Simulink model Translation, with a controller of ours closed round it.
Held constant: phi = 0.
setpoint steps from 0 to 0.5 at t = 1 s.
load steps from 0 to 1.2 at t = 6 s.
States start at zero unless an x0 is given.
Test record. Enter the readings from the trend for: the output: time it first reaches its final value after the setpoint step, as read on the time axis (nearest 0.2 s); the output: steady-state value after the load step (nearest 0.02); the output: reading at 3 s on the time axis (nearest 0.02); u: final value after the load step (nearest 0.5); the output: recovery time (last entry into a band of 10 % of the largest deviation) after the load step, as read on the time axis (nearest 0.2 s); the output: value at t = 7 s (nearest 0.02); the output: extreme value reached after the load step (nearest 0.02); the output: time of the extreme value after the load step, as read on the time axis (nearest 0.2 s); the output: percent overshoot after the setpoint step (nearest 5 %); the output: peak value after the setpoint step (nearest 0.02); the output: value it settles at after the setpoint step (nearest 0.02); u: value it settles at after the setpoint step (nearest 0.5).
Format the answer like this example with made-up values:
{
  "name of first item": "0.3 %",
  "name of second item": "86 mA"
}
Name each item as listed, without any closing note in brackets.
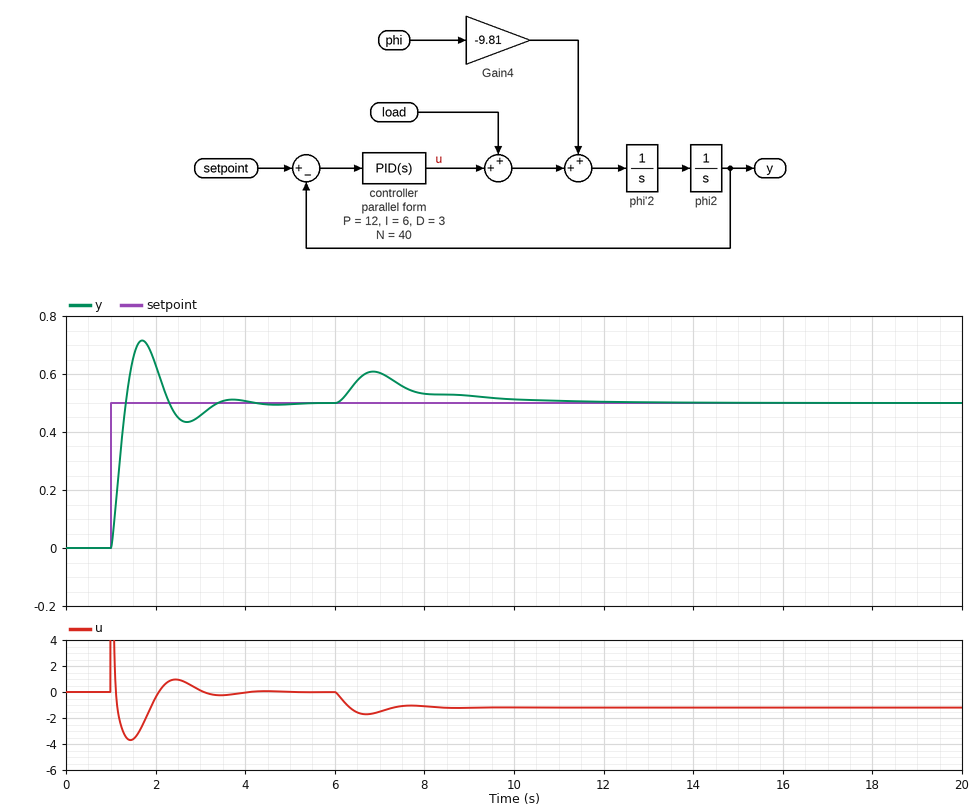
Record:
{
  "the output: time it first reaches its final value after the setpoint step, as read on the time axis": "1.4 s",
  "the output: steady-state value after the load step": "0.50",
  "the output: reading at 3 s on the time axis": "0.46",
  "u: final value after the load step": "-1.0",
  "the output: recovery time (last entry into a band of 10 % of the largest deviation) after the load step, as read on the time axis": "10.2 s",
  "the output: value at t = 7 s": "0.60",
  "the output: extreme value reached after the load step": "0.60",
  "the output: time of the extreme value after the load step, as read on the time axis": "6.8 s",
  "the output: percent overshoot after the setpoint step": "45 %",
  "the output: peak value after the setpoint step": "0.72",
  "the output: value it settles at after the setpoint step": "0.50",
  "u: value it settles at after the setpoint step": "0.0"
}
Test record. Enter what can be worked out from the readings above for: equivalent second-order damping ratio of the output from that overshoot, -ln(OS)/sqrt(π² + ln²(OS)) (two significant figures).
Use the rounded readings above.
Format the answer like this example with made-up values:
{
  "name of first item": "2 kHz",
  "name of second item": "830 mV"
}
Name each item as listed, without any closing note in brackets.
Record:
{
  "equivalent second-order damping ratio of the output from that overshoot, -ln(OS)/sqrt(π² + ln²(OS))": "0.25"
}
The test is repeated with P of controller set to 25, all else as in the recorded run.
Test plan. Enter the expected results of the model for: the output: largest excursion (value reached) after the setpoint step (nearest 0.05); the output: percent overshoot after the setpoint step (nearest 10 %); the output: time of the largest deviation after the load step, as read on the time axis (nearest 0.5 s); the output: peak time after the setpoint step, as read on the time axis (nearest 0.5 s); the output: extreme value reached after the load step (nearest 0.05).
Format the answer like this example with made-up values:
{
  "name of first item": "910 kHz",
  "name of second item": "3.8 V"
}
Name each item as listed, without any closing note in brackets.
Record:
{
  "the output: largest excursion (value reached) after the setpoint step": "0.75",
  "the output: percent overshoot after the setpoint step": "50 %",
  "the output: time of the largest deviation after the load step, as read on the time axis": "6.5 s",
  "the output: peak time after the setpoint step, as read on the time axis": "1.5 s",
  "the output: extreme value reached after the load step": "0.55"
}
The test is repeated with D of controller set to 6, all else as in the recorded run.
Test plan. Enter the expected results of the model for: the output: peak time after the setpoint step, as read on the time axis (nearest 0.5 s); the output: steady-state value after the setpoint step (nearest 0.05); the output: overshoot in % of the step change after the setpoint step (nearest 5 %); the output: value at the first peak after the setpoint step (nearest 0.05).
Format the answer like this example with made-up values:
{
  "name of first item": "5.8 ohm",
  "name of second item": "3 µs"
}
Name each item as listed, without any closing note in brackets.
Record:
{
  "the output: peak time after the setpoint step, as read on the time axis": "1.5 s",
  "the output: steady-state value after the setpoint step": "0.50",
  "the output: overshoot in % of the step change after the setpoint step": "20 %",
  "the output: value at the first peak after the setpoint step": "0.60"
}
